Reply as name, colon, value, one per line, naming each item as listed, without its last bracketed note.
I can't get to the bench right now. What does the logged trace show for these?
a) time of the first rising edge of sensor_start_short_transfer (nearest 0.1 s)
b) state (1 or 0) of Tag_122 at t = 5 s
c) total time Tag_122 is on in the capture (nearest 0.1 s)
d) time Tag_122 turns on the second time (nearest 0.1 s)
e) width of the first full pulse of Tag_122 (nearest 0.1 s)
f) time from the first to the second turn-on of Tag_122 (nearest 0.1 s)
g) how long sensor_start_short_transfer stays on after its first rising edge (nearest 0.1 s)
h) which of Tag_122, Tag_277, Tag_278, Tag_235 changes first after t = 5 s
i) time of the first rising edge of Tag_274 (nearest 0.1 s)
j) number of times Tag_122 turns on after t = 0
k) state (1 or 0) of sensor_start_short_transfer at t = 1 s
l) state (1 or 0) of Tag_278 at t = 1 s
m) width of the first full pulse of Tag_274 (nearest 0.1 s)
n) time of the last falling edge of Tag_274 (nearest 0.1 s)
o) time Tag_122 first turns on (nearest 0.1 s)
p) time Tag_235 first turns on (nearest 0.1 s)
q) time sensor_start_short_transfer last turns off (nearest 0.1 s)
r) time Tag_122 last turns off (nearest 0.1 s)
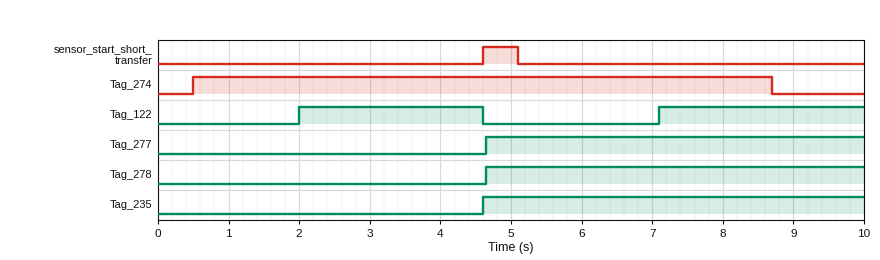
time of the first rising edge of sensor_start_short_transfer: 4.6 s
state (1 or 0) of Tag_122 at t = 5 s: 0
total time Tag_122 is on in the capture: 5.5 s
time Tag_122 turns on the second time: 7.1 s
width of the first full pulse of Tag_122: 2.6 s
time from the first to the second turn-on of Tag_122: 5.1 s
how long sensor_start_short_transfer stays on after its first rising edge: 0.5 s
which of Tag_122, Tag_277, Tag_278, Tag_235 changes first after t = 5 s: Tag_122
time of the first rising edge of Tag_274: 0.5 s
number of times Tag_122 turns on after t = 0: 2
state (1 or 0) of sensor_start_short_transfer at t = 1 s: 0
state (1 or 0) of Tag_278 at t = 1 s: 0
width of the first full pulse of Tag_274: 8.2 s
time of the last falling edge of Tag_274: 8.7 s
time Tag_122 first turns on: 2.0 s
time Tag_235 first turns on: 4.6 s
time sensor_start_short_transfer last turns off: 5.1 s
time Tag_122 last turns off: 4.6 s
